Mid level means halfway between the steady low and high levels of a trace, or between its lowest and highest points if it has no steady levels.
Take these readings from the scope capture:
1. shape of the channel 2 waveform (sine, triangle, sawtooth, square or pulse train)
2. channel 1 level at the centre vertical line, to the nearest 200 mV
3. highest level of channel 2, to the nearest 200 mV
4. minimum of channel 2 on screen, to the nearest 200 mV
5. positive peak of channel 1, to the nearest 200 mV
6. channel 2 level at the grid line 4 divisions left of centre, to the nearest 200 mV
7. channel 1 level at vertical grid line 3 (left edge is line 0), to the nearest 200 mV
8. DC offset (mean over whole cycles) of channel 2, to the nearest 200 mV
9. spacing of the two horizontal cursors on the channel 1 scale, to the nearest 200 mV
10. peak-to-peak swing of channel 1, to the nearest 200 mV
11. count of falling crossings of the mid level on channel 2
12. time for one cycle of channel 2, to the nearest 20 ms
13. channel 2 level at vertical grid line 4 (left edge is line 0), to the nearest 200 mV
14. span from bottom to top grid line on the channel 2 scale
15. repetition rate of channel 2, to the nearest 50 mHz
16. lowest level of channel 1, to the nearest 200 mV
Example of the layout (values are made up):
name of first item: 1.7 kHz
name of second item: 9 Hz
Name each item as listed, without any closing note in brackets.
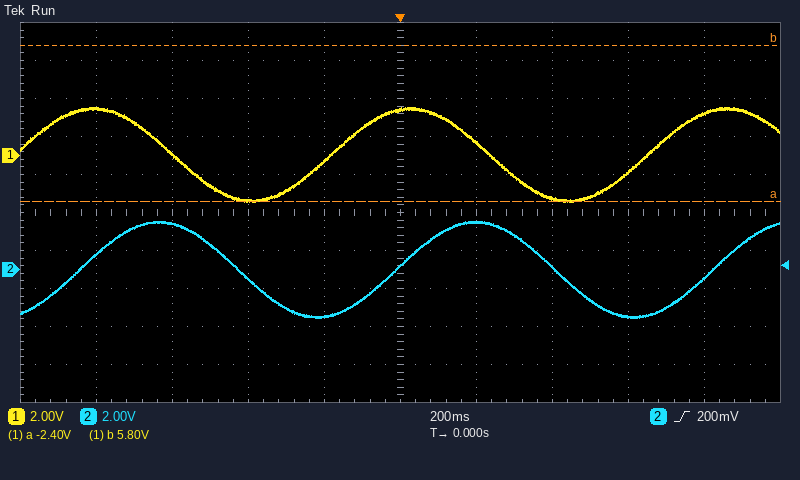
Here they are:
shape of the channel 2 waveform: sine
channel 1 level at the centre vertical line, to the nearest 200 mV: 2.4 V
highest level of channel 2, to the nearest 200 mV: 2.6 V
minimum of channel 2 on screen, to the nearest 200 mV: -2.6 V
positive peak of channel 1, to the nearest 200 mV: 2.6 V
channel 2 level at the grid line 4 divisions left of centre, to the nearest 200 mV: 800 mV
channel 1 level at vertical grid line 3 (left edge is line 0), to the nearest 200 mV: -2.4 V
DC offset (mean over whole cycles) of channel 2, to the nearest 200 mV: 0.0 V
spacing of the two horizontal cursors on the channel 1 scale, to the nearest 200 mV: 8.2 V
peak-to-peak swing of channel 1, to the nearest 200 mV: 5.0 V
count of falling crossings of the mid level on channel 2: 2
time for one cycle of channel 2, to the nearest 20 ms: 840 ms
channel 2 level at vertical grid line 4 (left edge is line 0), to the nearest 200 mV: -2.4 V
span from bottom to top grid line on the channel 2 scale: 20 V
repetition rate of channel 2, to the nearest 50 mHz: 1.20 Hz
lowest level of channel 1, to the nearest 200 mV: -2.4 V
